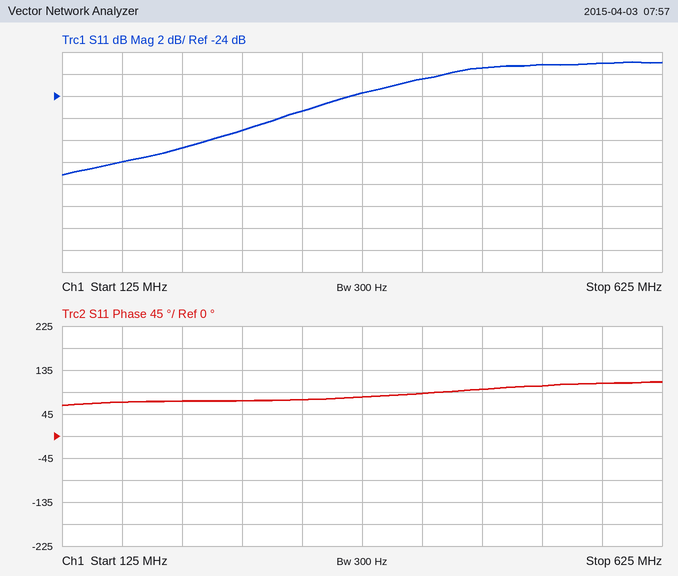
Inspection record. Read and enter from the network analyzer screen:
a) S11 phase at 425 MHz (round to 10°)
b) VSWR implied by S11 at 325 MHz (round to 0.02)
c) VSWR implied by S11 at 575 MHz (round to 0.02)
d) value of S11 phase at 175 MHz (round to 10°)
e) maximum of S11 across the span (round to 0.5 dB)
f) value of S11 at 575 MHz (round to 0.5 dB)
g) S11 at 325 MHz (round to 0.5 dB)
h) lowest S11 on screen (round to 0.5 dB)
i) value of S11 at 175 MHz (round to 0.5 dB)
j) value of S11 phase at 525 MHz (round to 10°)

90°
1.12
1.20
70°
-21.0 dB
-21.0 dB
-25.5 dB
-31.0 dB
-30.0 dB
100°
